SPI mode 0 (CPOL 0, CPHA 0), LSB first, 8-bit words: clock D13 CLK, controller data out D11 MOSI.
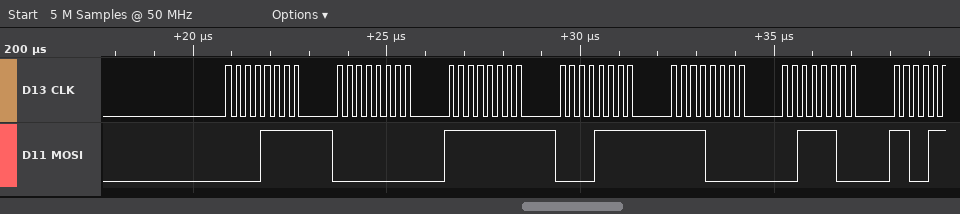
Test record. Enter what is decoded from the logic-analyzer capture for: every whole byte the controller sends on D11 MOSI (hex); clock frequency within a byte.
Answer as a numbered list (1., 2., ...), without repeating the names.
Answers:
1. F0 00 FF F0 0F 3C
2. 4 MHz
